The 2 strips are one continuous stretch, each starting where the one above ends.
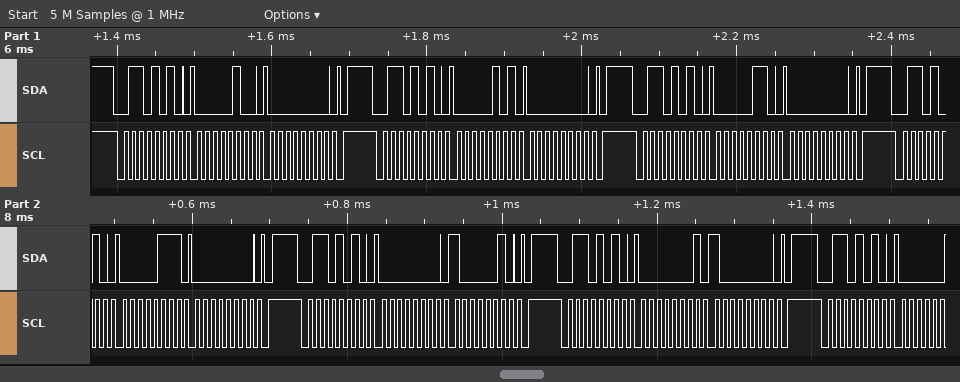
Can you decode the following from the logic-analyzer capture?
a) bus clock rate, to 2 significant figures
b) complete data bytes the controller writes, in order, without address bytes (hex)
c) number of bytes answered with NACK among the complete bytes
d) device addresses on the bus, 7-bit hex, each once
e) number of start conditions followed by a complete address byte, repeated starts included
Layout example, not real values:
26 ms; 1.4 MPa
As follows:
100 kHz; 04 00 05 00 06 00 07 00 00 82 01 80; 0; 0x35; 7
